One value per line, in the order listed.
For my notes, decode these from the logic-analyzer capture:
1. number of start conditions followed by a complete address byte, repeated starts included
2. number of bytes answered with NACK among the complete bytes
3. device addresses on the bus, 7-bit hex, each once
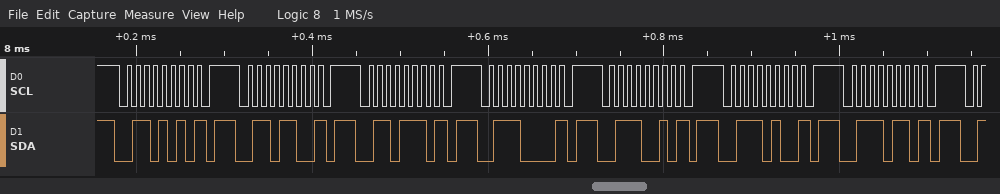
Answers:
7
7
0x35 0x36 0x37 0x38 0x39 0x3A 0x3B
